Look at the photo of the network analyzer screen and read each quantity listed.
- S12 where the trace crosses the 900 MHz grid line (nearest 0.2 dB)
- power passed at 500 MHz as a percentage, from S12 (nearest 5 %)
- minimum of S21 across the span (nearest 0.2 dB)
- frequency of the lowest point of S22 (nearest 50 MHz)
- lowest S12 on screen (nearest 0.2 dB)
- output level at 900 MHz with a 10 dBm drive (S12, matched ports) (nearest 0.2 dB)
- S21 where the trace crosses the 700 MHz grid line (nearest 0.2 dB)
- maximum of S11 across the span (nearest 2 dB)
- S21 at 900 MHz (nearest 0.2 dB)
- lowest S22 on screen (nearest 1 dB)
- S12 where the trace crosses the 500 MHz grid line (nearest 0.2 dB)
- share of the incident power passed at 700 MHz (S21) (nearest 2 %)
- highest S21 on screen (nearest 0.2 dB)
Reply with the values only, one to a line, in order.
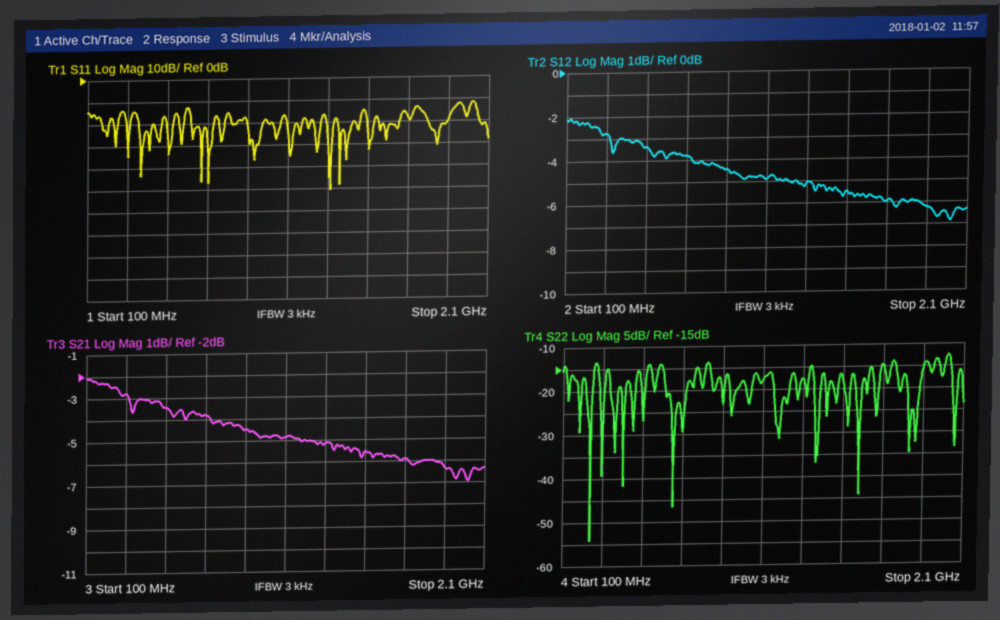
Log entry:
-4.4 dB
45 %
-7.0 dB
250 MHz
-6.8 dB
5.6 dBm
-3.8 dB
-12 dB
-4.4 dB
-54 dB
-3.4 dB
42 %
-2.0 dB
